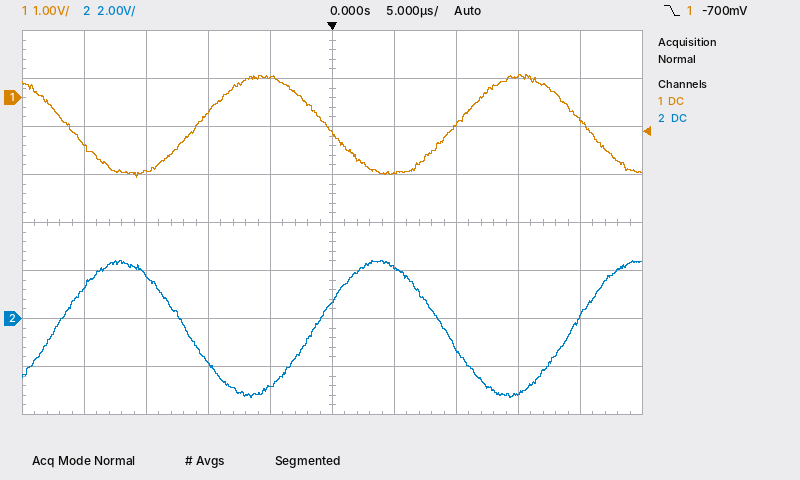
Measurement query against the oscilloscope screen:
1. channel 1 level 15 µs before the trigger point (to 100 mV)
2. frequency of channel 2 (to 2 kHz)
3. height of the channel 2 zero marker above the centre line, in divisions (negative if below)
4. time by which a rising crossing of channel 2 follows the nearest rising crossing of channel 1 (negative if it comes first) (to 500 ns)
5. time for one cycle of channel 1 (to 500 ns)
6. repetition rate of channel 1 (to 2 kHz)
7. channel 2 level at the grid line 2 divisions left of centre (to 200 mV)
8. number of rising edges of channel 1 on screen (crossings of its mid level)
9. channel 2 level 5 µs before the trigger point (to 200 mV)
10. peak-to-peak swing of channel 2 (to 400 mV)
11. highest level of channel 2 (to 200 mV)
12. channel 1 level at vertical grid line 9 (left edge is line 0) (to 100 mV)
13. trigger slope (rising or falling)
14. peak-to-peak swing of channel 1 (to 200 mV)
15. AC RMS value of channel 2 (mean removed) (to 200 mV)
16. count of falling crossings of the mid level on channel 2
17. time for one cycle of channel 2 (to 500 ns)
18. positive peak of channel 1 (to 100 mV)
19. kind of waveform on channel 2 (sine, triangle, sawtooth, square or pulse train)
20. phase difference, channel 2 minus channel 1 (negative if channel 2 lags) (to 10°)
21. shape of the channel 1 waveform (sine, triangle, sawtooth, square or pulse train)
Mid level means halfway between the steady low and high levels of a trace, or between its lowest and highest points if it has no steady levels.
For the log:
-1.5 V
48 kHz
-2.0 div
+9.5 µs
21.0 µs
48 kHz
-1.8 V
2
-2.8 V
5.6 V
2.4 V
-500 mV
falling
2.2 V
2.0 V
2
21.0 µs
500 mV
sine
-160°
sine
